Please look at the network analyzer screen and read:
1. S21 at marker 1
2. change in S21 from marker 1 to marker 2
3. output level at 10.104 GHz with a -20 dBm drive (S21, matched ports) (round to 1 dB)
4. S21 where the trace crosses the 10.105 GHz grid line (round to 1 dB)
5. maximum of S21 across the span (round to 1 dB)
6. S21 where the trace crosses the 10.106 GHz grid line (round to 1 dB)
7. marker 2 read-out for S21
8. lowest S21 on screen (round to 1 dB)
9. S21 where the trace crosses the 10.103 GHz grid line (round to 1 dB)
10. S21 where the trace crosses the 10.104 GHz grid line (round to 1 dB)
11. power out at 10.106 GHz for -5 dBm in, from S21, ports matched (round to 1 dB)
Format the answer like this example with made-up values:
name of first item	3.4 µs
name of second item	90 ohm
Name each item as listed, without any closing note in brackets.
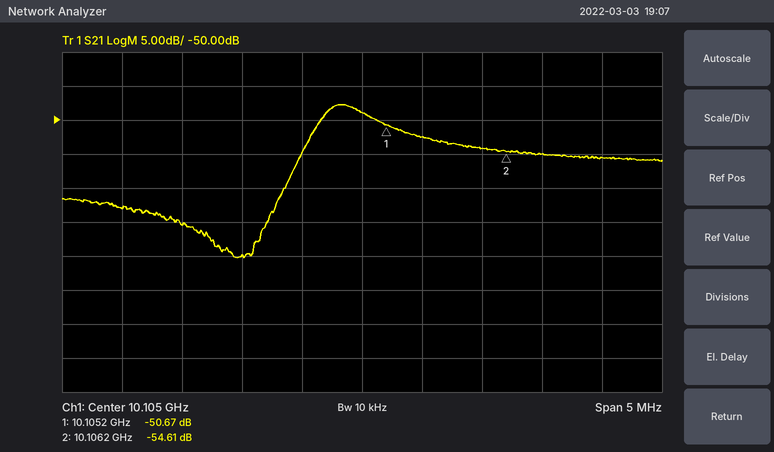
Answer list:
S21 at marker 1	-50.67 dB
change in S21 from marker 1 to marker 2	-3.94 dB
output level at 10.104 GHz with a -20 dBm drive (S21, matched ports)	-90 dBm
S21 where the trace crosses the 10.105 GHz grid line	-49 dB
maximum of S21 across the span	-48 dB
S21 where the trace crosses the 10.106 GHz grid line	-54 dB
marker 2 read-out for S21	-54.61 dB
lowest S21 on screen	-70 dB
S21 where the trace crosses the 10.103 GHz grid line	-63 dB
S21 where the trace crosses the 10.104 GHz grid line	-70 dB
power out at 10.106 GHz for -5 dBm in, from S21, ports matched	-59 dBm
